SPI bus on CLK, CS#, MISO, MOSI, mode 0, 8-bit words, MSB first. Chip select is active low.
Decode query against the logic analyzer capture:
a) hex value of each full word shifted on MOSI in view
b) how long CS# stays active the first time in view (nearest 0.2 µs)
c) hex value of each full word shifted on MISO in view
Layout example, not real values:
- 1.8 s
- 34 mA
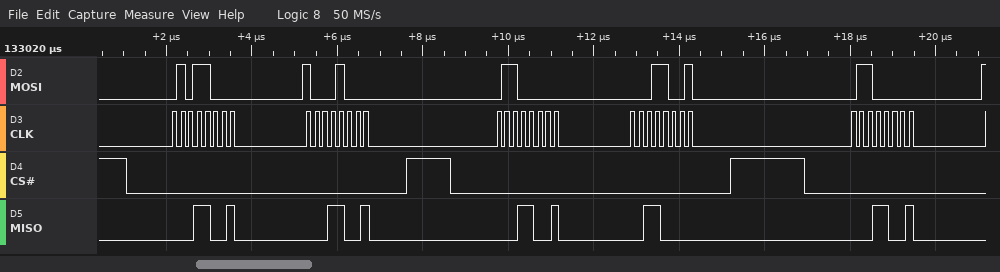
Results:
- 58, 88, 60, 19, 60
- 6.6 µs
- 19, 19, 19, 30, 19
